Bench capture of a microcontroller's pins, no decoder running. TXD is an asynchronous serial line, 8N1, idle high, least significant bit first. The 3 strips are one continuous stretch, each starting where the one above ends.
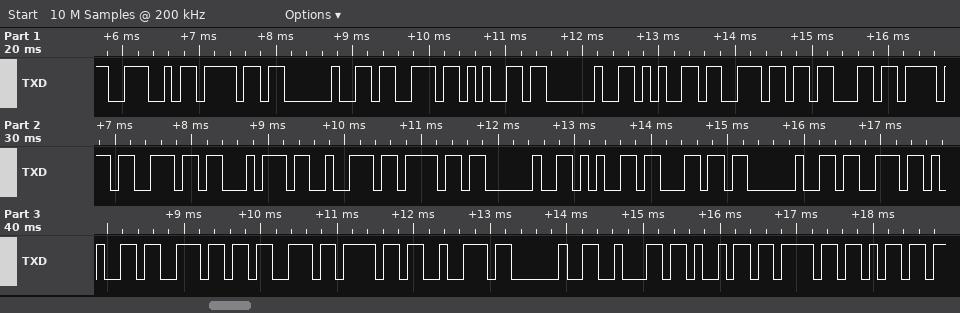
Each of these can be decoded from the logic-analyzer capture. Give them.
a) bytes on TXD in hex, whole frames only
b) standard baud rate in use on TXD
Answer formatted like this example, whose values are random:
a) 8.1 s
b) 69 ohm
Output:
a) 4E 6F 20 73 65 20 65 6E 63 6F 6E 74 72 6F 20 65 6C 20 73 65 6E 73 6F 72 20 62 69 6F 6D
b) 9600 baud
